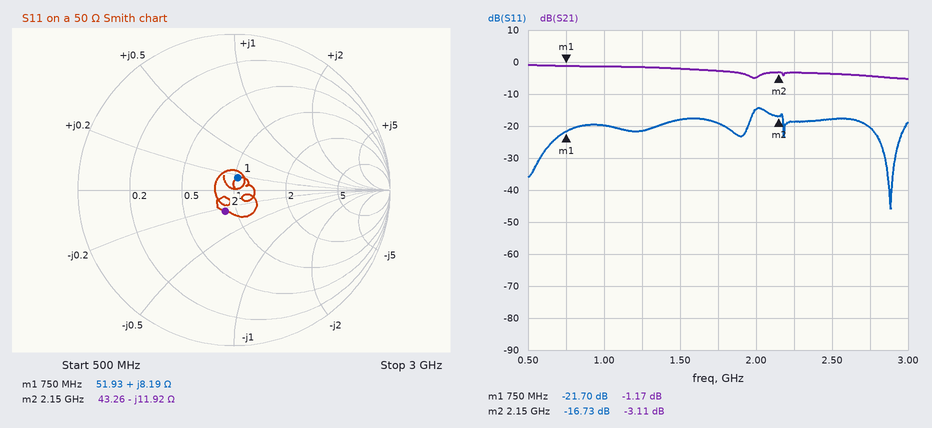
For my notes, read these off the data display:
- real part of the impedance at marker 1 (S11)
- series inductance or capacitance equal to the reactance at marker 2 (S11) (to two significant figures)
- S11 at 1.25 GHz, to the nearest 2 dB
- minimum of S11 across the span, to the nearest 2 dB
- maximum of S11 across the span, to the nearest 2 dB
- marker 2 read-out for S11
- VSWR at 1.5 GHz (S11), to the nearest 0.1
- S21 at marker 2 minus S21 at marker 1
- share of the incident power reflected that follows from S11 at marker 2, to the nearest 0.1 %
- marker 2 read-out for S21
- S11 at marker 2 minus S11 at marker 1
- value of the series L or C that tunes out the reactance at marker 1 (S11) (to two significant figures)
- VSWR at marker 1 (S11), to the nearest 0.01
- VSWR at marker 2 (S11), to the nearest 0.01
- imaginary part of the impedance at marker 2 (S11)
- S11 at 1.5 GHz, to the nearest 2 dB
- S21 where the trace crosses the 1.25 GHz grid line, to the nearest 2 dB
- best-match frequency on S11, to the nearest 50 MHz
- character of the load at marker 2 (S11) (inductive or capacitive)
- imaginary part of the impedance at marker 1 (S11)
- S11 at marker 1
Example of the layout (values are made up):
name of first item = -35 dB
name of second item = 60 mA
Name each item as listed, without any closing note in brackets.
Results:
real part of the impedance at marker 1 = 51.93 Ω
series inductance or capacitance equal to the reactance at marker 2 (S11) = 6.2 pF
S11 at 1.25 GHz, to the nearest 2 dB = -22 dB
minimum of S11 across the span, to the nearest 2 dB = -46 dB
maximum of S11 across the span, to the nearest 2 dB = -14 dB
marker 2 read-out for S11 = -16.73 dB
VSWR at 1.5 GHz (S11), to the nearest 0.1 = 1.3
S21 at marker 2 minus S21 at marker 1 = -1.94 dB
share of the incident power reflected that follows from S11 at marker 2, to the nearest 0.1 % = 2.1 %
marker 2 read-out for S21 = -3.11 dB
S11 at marker 2 minus S11 at marker 1 = 4.97 dB
value of the series L or C that tunes out the reactance at marker 1 (S11) = 26 pF
VSWR at marker 1 (S11), to the nearest 0.01 = 1.18
VSWR at marker 2 (S11), to the nearest 0.01 = 1.34
imaginary part of the impedance at marker 2 = -11.92 Ω
S11 at 1.5 GHz, to the nearest 2 dB = -18 dB
S21 where the trace crosses the 1.25 GHz grid line, to the nearest 2 dB = -2 dB
best-match frequency on S11, to the nearest 50 MHz = 2.90 GHz
character of the load at marker 2 (S11) = capacitive
imaginary part of the impedance at marker 1 = +8.19 Ω
S11 at marker 1 = -21.70 dB
